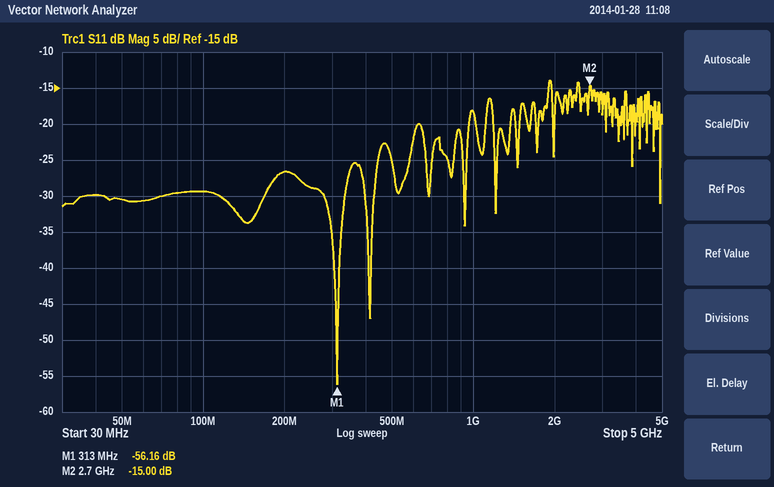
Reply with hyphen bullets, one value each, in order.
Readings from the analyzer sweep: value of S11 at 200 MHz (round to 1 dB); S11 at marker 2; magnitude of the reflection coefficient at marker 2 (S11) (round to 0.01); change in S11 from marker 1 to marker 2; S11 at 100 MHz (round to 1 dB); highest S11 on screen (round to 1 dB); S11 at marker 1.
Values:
- -27 dB
- -15.00 dB
- 0.18
- 41.16 dB
- -29 dB
- -14 dB
- -56.16 dB
